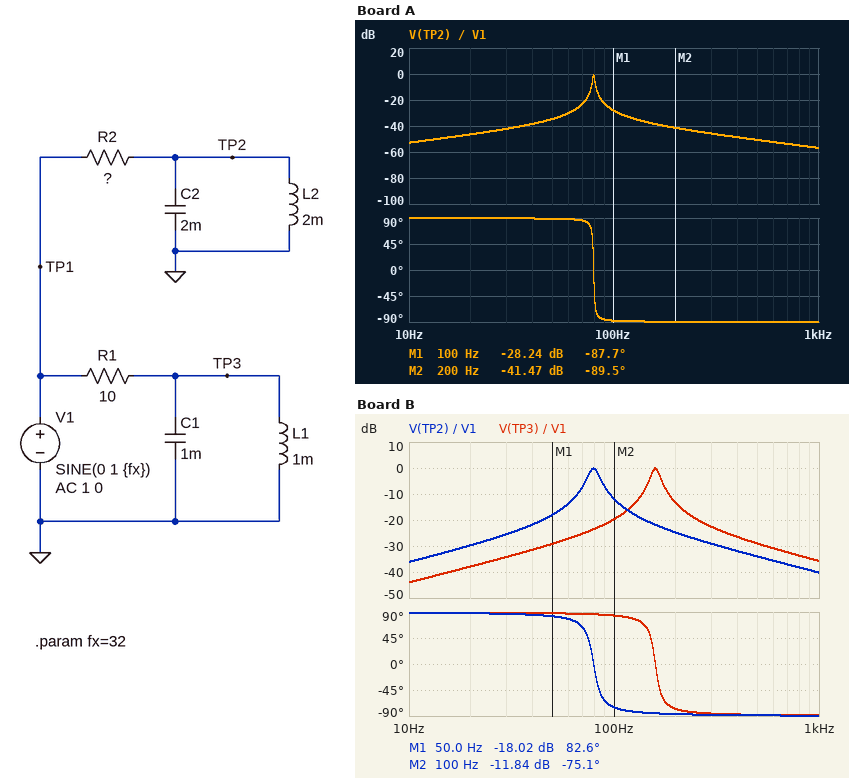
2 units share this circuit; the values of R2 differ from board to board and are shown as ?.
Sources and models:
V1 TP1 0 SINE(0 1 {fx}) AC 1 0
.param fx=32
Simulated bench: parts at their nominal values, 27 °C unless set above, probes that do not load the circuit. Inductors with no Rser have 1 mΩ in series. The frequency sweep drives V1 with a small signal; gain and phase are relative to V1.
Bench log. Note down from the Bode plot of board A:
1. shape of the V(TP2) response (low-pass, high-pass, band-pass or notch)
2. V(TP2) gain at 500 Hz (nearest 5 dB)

band-pass
-50 dB
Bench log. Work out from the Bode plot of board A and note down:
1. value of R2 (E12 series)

56 Ω
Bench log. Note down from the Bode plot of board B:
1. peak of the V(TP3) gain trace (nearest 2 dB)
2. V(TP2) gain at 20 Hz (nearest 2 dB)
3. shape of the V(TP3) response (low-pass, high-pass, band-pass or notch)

0 dB
-30 dB
band-pass
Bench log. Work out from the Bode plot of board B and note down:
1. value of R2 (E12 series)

8.2 Ω
